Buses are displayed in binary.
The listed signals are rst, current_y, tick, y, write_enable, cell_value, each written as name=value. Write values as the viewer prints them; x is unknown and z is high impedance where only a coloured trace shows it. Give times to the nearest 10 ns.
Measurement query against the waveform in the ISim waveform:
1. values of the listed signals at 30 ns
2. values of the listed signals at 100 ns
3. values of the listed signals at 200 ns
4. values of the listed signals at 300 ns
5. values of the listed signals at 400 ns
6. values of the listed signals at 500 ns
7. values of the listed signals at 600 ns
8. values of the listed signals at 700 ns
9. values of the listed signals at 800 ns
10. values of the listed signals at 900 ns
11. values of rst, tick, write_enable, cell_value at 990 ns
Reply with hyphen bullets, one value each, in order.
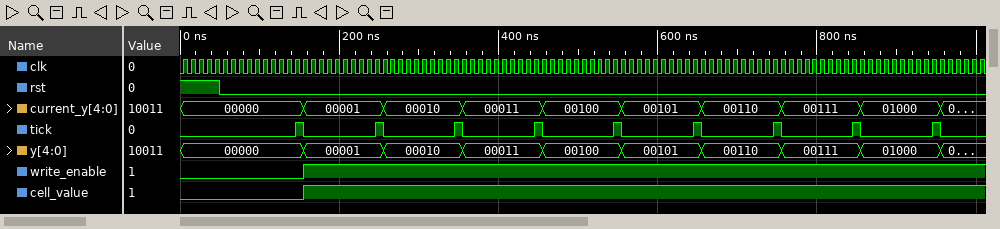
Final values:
- rst=1, current_y=00000, tick=0, y=00000, write_enable=0, cell_value=0
- rst=0, current_y=00000, tick=0, y=00000, write_enable=0, cell_value=0
- rst=0, current_y=00001, tick=0, y=00001, write_enable=1, cell_value=1
- rst=0, current_y=00010, tick=0, y=00010, write_enable=1, cell_value=1
- rst=0, current_y=00011, tick=0, y=00011, write_enable=1, cell_value=1
- rst=0, current_y=00100, tick=0, y=00100, write_enable=1, cell_value=1
- rst=0, current_y=00101, tick=0, y=00101, write_enable=1, cell_value=1
- rst=0, current_y=00110, tick=0, y=00110, write_enable=1, cell_value=1
- rst=0, current_y=00111, tick=0, y=00111, write_enable=1, cell_value=1
- rst=0, current_y=01000, tick=0, y=01000, write_enable=1, cell_value=1
- rst=0, tick=0, write_enable=1, cell_value=1
